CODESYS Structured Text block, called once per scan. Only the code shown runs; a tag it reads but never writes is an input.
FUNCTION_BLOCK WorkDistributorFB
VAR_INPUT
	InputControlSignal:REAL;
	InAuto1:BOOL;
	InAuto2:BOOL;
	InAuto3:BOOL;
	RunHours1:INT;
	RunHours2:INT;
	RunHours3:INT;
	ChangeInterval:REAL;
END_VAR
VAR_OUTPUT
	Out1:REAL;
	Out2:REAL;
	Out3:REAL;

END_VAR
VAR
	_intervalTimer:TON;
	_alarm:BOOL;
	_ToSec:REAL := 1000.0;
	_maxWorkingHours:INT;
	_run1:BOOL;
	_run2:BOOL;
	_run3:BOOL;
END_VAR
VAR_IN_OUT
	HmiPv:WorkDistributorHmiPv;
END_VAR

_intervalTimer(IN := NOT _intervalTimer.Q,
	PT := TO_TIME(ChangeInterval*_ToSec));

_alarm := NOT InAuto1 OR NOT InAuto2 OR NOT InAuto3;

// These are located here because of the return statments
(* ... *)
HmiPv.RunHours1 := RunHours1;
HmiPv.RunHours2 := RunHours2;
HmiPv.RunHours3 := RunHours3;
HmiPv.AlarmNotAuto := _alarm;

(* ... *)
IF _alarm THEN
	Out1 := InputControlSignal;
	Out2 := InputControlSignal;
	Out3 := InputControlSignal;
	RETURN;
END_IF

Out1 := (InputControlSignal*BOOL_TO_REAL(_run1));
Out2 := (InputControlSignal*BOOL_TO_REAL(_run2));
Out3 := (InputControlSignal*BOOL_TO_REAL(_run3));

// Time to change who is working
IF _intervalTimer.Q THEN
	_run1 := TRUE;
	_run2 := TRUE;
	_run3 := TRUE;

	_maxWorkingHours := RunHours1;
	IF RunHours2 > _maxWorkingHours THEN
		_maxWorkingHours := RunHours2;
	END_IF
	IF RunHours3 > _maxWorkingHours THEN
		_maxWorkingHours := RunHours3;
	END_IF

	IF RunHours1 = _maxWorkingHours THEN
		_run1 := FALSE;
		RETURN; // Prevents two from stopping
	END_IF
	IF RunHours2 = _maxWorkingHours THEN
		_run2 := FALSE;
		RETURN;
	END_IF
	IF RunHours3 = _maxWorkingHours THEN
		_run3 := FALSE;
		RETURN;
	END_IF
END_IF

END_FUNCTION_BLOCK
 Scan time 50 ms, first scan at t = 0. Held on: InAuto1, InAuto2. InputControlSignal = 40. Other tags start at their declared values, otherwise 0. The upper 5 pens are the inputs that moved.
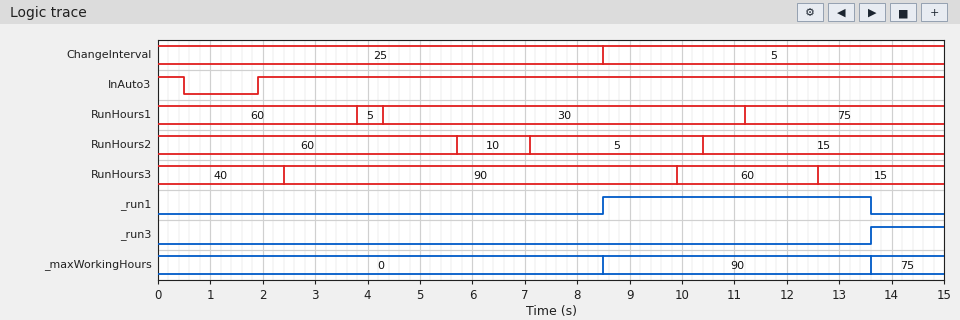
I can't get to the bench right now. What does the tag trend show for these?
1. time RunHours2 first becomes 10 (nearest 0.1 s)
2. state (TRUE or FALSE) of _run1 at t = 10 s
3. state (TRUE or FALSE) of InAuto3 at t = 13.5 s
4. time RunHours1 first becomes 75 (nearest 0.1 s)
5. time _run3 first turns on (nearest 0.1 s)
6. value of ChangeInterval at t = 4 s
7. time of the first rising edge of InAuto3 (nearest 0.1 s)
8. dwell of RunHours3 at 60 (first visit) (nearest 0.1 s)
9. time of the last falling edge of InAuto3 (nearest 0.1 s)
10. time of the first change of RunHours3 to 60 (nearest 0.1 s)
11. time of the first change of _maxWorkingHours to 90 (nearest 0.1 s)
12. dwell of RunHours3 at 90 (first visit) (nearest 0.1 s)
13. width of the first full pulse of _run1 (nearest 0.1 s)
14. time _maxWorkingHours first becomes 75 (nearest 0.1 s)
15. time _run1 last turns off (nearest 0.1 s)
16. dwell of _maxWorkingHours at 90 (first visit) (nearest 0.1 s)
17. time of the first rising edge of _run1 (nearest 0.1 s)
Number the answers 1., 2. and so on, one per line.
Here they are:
1. 5.7 s
2. TRUE
3. TRUE
4. 11.2 s
5. 13.6 s
6. 25
7. 1.9 s
8. 2.7 s
9. 0.5 s
10. 9.9 s
11. 8.5 s
12. 7.5 s
13. 5.1 s
14. 13.6 s
15. 13.6 s
16. 5.1 s
17. 8.5 s
